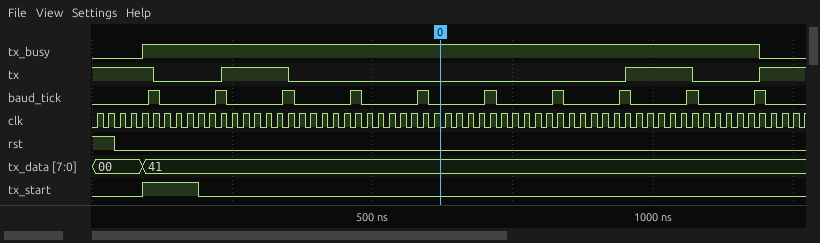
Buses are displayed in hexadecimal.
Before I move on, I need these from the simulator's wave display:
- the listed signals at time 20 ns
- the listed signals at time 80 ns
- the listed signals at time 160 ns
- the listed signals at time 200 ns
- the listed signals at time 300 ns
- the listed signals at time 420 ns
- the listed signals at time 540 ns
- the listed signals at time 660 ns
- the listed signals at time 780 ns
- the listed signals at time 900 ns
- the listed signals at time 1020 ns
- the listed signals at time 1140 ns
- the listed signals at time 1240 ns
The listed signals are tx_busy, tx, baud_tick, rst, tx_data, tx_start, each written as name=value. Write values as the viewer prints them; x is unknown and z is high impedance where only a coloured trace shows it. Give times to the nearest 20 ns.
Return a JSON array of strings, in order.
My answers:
["tx_busy=0, tx=1, baud_tick=0, rst=1, tx_data=00, tx_start=0", "tx_busy=0, tx=1, baud_tick=0, rst=0, tx_data=00, tx_start=0", "tx_busy=1, tx=0, baud_tick=0, rst=0, tx_data=41, tx_start=1", "tx_busy=1, tx=0, baud_tick=0, rst=0, tx_data=41, tx_start=0", "tx_busy=1, tx=1, baud_tick=0, rst=0, tx_data=41, tx_start=0", "tx_busy=1, tx=0, baud_tick=0, rst=0, tx_data=41, tx_start=0", "tx_busy=1, tx=0, baud_tick=0, rst=0, tx_data=41, tx_start=0", "tx_busy=1, tx=0, baud_tick=0, rst=0, tx_data=41, tx_start=0", "tx_busy=1, tx=0, baud_tick=0, rst=0, tx_data=41, tx_start=0", "tx_busy=1, tx=0, baud_tick=0, rst=0, tx_data=41, tx_start=0", "tx_busy=1, tx=1, baud_tick=0, rst=0, tx_data=41, tx_start=0", "tx_busy=1, tx=0, baud_tick=0, rst=0, tx_data=41, tx_start=0", "tx_busy=0, tx=1, baud_tick=0, rst=0, tx_data=41, tx_start=0"]
